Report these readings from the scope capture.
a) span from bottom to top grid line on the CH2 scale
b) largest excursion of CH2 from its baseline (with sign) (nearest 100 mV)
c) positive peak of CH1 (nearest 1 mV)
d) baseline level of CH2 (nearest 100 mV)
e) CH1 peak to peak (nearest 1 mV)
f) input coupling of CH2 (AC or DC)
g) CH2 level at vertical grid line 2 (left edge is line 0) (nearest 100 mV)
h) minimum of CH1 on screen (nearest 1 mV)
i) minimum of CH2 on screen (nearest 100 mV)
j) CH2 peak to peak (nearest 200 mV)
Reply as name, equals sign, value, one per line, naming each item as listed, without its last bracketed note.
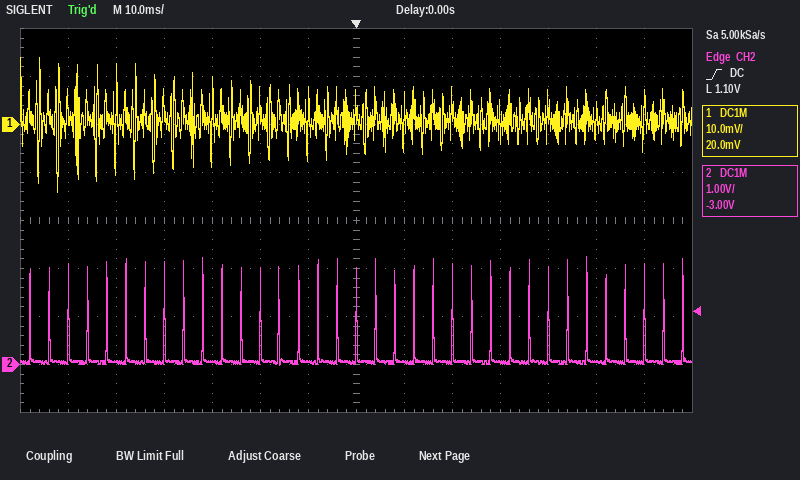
span from bottom to top grid line on the CH2 scale = 8 V
largest excursion of CH2 from its baseline (with sign) = +2.2 V
positive peak of CH1 = 14 mV
baseline level of CH2 = 100 mV
CH1 peak to peak = 28 mV
input coupling of CH2 = DC
CH2 level at vertical grid line 2 (left edge is line 0) = 100 mV
minimum of CH1 on screen = -14 mV
minimum of CH2 on screen = 0.0 V
CH2 peak to peak = 2.2 V
